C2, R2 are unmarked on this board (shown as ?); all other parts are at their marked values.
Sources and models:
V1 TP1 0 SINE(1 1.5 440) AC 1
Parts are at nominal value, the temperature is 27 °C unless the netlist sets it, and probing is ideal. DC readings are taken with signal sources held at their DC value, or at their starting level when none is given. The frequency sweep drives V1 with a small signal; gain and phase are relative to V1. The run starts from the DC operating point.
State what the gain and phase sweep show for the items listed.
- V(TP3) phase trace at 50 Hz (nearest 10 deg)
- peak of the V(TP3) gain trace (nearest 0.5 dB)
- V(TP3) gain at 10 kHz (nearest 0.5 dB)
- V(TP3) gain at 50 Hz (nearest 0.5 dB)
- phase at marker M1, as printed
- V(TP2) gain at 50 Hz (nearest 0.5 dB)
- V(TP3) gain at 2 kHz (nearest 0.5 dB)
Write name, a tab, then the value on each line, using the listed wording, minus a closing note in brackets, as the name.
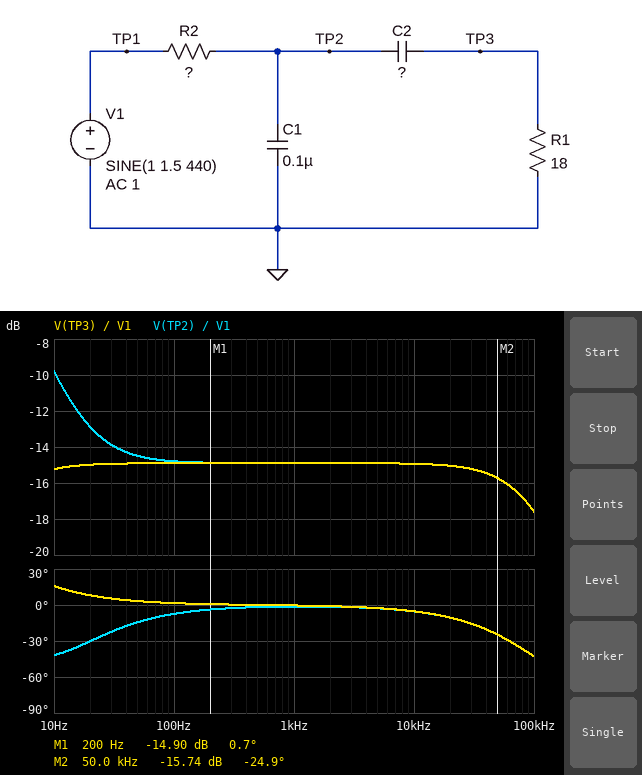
V(TP3) phase trace at 50 Hz	0 deg
peak of the V(TP3) gain trace	-15.0 dB
V(TP3) gain at 10 kHz	-15.0 dB
V(TP3) gain at 50 Hz	-15.0 dB
phase at marker M1, as printed	0.7 deg
V(TP2) gain at 50 Hz	-14.5 dB
V(TP3) gain at 2 kHz	-15.0 dB
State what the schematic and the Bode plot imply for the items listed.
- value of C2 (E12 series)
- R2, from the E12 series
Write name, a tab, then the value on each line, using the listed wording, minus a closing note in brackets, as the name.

value of C2	560 µF
R2, from the E12 series	82 Ω
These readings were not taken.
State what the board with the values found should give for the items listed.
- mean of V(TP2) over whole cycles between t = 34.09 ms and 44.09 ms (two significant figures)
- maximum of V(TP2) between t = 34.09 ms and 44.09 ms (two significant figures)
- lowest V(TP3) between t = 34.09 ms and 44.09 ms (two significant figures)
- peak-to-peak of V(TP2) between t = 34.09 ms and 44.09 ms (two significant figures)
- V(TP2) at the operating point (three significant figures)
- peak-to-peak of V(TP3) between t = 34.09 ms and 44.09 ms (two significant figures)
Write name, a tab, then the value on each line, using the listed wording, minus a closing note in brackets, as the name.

mean of V(TP2) over whole cycles between t = 34.09 ms and 44.09 ms	1.0 V
maximum of V(TP2) between t = 34.09 ms and 44.09 ms	1.3 V
lowest V(TP3) between t = 34.09 ms and 44.09 ms	-270 mV
peak-to-peak of V(TP2) between t = 34.09 ms and 44.09 ms	540 mV
V(TP2) at the operating point	1.00 V
peak-to-peak of V(TP3) between t = 34.09 ms and 44.09 ms	540 mV
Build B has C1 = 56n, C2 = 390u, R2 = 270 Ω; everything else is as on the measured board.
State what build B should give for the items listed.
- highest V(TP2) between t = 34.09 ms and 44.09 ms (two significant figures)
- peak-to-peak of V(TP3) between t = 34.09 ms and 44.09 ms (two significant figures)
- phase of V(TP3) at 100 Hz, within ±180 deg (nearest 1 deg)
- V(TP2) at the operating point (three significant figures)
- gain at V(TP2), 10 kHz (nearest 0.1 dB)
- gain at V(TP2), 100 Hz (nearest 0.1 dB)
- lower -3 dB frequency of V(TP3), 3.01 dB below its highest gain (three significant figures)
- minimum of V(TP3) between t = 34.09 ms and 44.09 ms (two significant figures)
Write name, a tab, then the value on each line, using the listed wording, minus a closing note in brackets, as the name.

highest V(TP2) between t = 34.09 ms and 44.09 ms	1.1 V
peak-to-peak of V(TP3) between t = 34.09 ms and 44.09 ms	190 mV
phase of V(TP3) at 100 Hz, within ±180 deg	1 deg
V(TP2) at the operating point	1.00 V
gain at V(TP2), 10 kHz	-24.1 dB
gain at V(TP2), 100 Hz	-23.9 dB
lower -3 dB frequency of V(TP3), 3.01 dB below its highest gain	1.42 Hz
minimum of V(TP3) between t = 34.09 ms and 44.09 ms	-94 mV
